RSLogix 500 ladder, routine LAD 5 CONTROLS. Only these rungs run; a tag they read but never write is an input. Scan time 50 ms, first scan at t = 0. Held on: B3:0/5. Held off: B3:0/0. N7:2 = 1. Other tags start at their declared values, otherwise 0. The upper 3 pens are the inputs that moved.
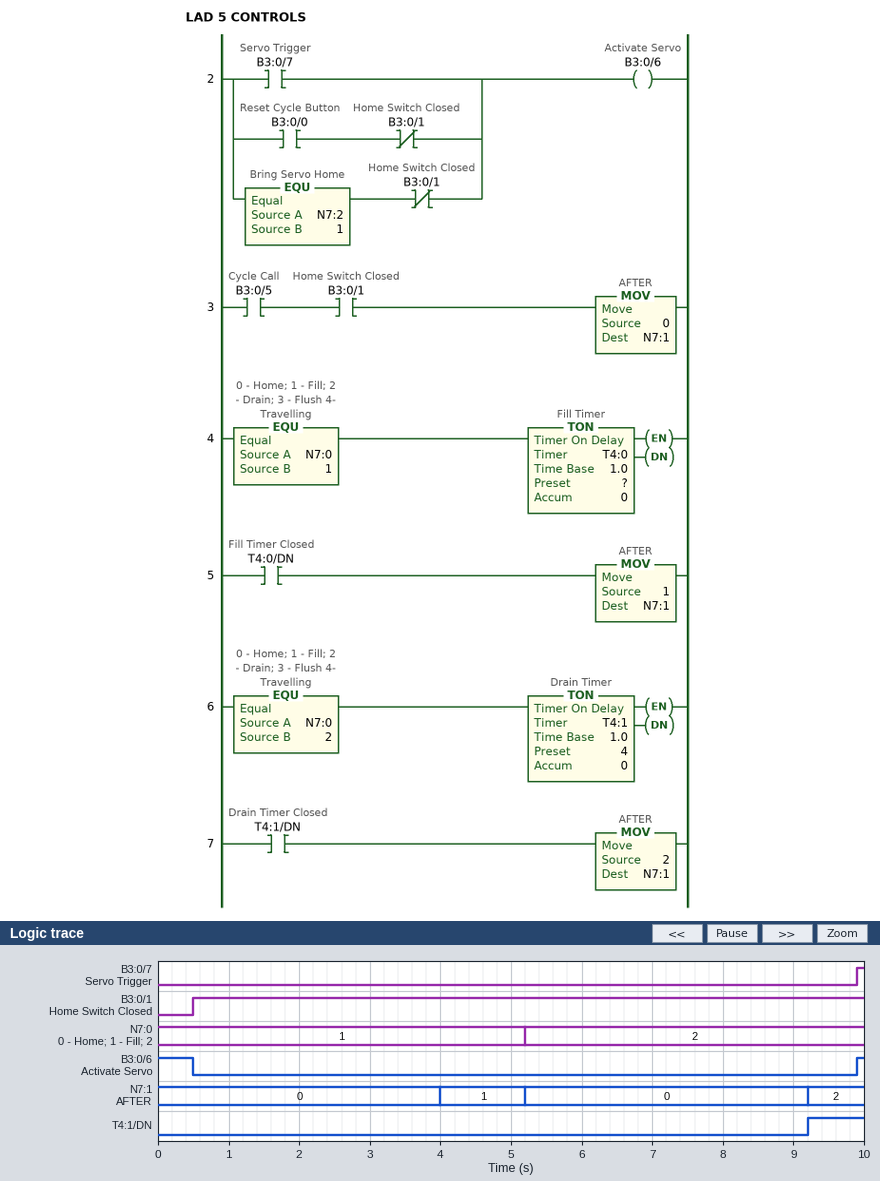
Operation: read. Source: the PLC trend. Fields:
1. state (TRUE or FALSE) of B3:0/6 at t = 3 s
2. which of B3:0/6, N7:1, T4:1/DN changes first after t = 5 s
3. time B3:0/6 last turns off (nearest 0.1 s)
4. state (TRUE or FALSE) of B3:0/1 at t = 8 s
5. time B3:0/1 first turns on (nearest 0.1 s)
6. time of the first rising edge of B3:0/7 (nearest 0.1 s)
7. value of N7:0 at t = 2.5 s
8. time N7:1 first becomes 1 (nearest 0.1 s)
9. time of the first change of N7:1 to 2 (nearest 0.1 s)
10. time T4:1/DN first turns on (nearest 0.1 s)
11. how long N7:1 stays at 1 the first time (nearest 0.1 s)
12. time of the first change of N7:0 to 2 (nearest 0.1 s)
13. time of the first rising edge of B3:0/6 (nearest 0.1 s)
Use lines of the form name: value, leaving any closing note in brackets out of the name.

state (TRUE or FALSE) of B3:0/6 at t = 3 s: FALSE
which of B3:0/6, N7:1, T4:1/DN changes first after t = 5 s: N7:1
time B3:0/6 last turns off: 0.5 s
state (TRUE or FALSE) of B3:0/1 at t = 8 s: TRUE
time B3:0/1 first turns on: 0.5 s
time of the first rising edge of B3:0/7: 9.9 s
value of N7:0 at t = 2.5 s: 1
time N7:1 first becomes 1: 4.0 s
time of the first change of N7:1 to 2: 9.2 s
time T4:1/DN first turns on: 9.2 s
how long N7:1 stays at 1 the first time: 1.2 s
time of the first change of N7:0 to 2: 5.2 s
time of the first rising edge of B3:0/6: 9.9 s
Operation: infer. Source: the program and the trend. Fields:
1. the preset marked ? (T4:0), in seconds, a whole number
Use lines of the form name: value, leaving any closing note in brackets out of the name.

the preset marked ? (T4:0), in seconds, a whole number: 4 s
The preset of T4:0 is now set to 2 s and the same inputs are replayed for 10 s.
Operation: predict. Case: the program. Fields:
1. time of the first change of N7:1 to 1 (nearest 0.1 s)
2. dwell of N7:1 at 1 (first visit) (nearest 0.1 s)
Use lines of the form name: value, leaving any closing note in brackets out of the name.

time of the first change of N7:1 to 1: 2.0 s
dwell of N7:1 at 1 (first visit): 3.2 s
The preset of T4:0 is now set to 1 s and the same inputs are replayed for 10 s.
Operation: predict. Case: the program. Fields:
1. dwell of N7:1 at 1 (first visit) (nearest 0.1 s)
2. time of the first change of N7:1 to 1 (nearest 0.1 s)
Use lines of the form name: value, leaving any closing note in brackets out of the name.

dwell of N7:1 at 1 (first visit): 4.2 s
time of the first change of N7:1 to 1: 1.0 s
